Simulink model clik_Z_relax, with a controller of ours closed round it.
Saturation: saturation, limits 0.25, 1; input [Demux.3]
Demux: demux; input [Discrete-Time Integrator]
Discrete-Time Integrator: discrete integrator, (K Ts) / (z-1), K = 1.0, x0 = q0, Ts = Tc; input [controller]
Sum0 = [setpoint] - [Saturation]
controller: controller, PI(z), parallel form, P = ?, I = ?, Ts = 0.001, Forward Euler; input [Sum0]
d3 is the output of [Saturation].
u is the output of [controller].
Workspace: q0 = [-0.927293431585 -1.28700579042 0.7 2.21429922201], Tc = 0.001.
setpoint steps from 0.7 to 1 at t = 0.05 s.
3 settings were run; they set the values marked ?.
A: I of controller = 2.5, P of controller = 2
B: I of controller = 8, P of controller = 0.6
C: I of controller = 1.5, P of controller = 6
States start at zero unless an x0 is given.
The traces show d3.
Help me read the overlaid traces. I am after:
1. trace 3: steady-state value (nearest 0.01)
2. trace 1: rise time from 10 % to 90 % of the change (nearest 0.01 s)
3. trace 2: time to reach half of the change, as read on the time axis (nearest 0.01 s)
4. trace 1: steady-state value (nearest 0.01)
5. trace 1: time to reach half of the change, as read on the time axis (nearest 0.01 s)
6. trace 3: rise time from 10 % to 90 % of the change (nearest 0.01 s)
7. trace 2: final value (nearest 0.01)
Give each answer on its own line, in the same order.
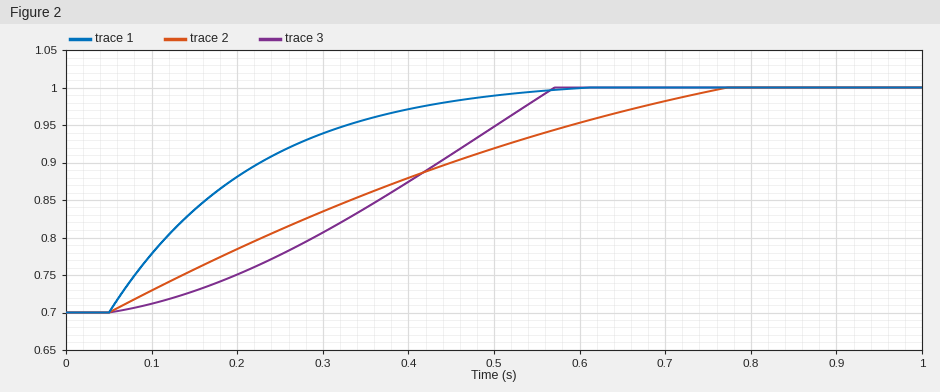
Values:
1.00
0.33 s
0.33 s
1.00
0.16 s
0.38 s
1.00
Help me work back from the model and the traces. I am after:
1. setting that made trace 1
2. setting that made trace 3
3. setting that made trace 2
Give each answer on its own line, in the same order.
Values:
C
B
A
